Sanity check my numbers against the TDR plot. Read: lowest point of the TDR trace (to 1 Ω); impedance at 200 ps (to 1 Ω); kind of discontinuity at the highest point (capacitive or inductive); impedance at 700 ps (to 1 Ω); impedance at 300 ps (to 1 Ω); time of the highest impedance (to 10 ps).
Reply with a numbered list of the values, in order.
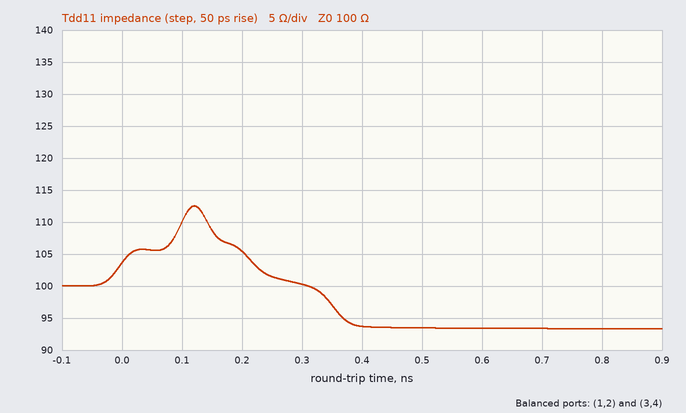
1. 93 Ω
2. 105 Ω
3. inductive
4. 93 Ω
5. 100 Ω
6. 120 ps
